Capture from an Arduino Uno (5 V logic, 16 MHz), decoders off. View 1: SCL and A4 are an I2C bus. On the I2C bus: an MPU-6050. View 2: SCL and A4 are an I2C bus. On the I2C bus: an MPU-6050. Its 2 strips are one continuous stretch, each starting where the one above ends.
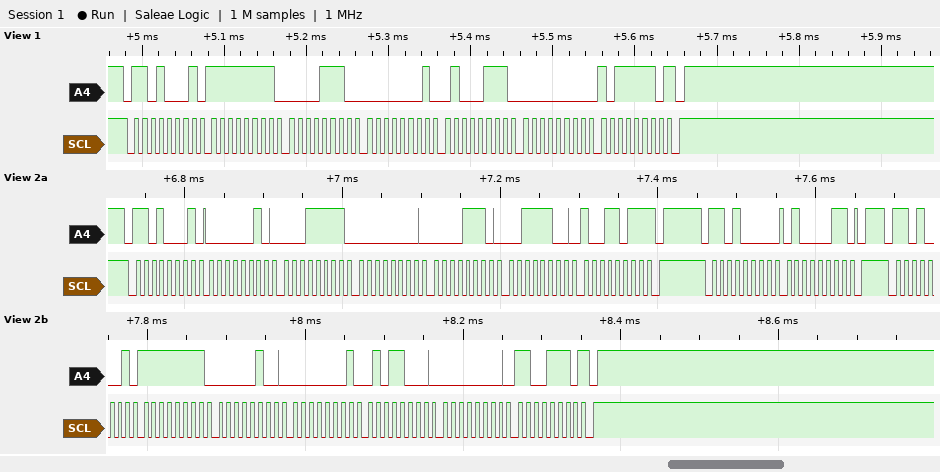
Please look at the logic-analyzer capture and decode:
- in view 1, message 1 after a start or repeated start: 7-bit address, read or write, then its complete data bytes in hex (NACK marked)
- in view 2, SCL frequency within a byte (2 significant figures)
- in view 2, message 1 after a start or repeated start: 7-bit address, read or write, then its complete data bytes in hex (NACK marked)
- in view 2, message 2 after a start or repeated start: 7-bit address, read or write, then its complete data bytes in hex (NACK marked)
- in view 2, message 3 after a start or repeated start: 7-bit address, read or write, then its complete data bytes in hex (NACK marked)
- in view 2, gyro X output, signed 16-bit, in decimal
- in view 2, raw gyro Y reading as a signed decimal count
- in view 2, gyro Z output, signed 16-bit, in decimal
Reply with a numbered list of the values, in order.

1. 0x68 read: FF 0E 01 47 00 BE NACK
2. 100 kHz
3. 0x68 read: 02 1F 00 0E 3C 9B NACK
4. 0x68 write: 43
5. 0x68 read: FF 04 01 58 00 CE NACK
6. -252
7. 344
8. 206
